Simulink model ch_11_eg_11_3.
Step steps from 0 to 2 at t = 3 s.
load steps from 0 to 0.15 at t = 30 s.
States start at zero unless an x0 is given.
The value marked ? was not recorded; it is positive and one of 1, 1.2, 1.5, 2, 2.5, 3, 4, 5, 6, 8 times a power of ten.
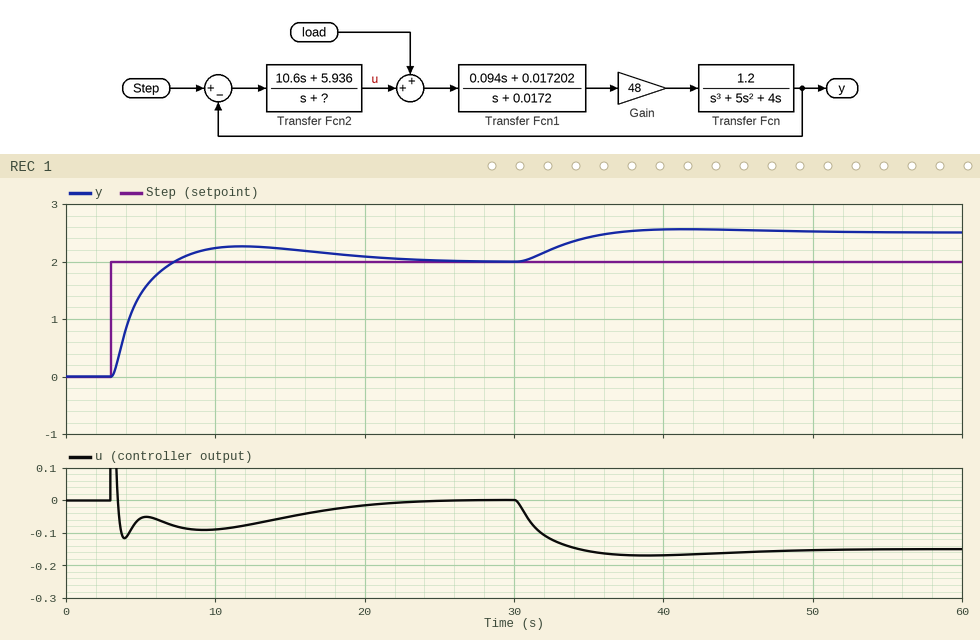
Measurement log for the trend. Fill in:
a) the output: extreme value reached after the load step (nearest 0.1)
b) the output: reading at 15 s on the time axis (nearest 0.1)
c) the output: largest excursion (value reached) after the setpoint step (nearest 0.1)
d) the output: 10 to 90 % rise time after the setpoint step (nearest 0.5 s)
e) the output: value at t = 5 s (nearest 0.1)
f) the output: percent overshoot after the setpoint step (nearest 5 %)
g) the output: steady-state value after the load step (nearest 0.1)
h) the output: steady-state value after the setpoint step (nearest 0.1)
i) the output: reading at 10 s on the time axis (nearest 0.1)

2.6
2.2
2.3
3.0 s
1.4
15 %
2.5
2.0
2.2
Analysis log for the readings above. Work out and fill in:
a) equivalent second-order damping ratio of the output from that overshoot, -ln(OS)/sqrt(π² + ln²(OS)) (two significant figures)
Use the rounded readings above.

0.52
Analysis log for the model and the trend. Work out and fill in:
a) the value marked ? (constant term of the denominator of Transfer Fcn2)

20
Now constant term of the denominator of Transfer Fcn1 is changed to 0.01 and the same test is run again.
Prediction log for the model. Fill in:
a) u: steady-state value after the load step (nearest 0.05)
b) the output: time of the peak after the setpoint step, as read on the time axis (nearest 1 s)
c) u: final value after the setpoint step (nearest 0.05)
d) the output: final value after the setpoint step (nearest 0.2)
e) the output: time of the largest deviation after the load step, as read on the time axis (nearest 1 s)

-0.15
12 s
0.00
2.0
41 s
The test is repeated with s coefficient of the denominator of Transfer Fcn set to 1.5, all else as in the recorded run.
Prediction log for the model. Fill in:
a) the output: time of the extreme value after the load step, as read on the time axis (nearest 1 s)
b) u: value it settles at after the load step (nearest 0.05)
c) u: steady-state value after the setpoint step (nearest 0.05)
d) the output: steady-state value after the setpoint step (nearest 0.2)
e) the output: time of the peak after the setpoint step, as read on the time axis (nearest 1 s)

37 s
-0.15
0.00
2.0
7 s
